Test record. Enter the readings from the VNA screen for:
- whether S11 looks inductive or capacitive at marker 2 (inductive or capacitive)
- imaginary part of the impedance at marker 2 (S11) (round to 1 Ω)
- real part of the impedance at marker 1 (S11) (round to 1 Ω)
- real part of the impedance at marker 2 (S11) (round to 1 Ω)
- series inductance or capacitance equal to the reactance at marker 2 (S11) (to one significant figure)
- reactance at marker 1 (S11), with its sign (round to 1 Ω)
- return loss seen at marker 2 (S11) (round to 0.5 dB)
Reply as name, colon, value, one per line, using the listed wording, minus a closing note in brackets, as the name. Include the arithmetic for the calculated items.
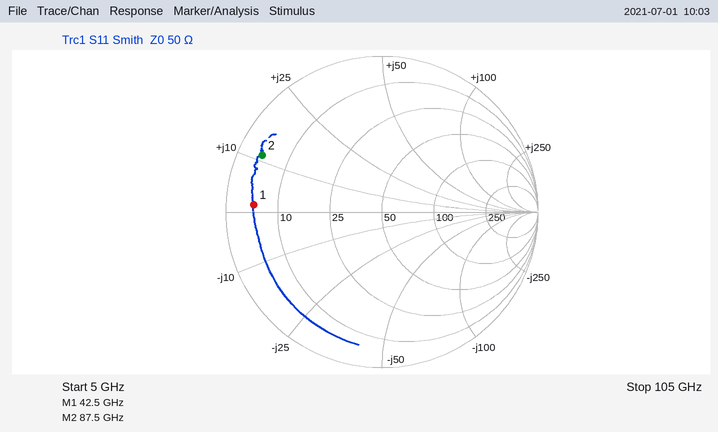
whether S11 looks inductive or capacitive at marker 2: inductive
imaginary part of the impedance at marker 2 (S11): +11 Ω
real part of the impedance at marker 1 (S11): 5 Ω
real part of the impedance at marker 2 (S11): 4 Ω
series inductance or capacitance equal to the reactance at marker 2 (S11): L = 11 Ω/(2π × 87.5 GHz) ≈ 20 pH
reactance at marker 1 (S11), with its sign: +1 Ω
return loss seen at marker 2 (S11): 1.5 dB
